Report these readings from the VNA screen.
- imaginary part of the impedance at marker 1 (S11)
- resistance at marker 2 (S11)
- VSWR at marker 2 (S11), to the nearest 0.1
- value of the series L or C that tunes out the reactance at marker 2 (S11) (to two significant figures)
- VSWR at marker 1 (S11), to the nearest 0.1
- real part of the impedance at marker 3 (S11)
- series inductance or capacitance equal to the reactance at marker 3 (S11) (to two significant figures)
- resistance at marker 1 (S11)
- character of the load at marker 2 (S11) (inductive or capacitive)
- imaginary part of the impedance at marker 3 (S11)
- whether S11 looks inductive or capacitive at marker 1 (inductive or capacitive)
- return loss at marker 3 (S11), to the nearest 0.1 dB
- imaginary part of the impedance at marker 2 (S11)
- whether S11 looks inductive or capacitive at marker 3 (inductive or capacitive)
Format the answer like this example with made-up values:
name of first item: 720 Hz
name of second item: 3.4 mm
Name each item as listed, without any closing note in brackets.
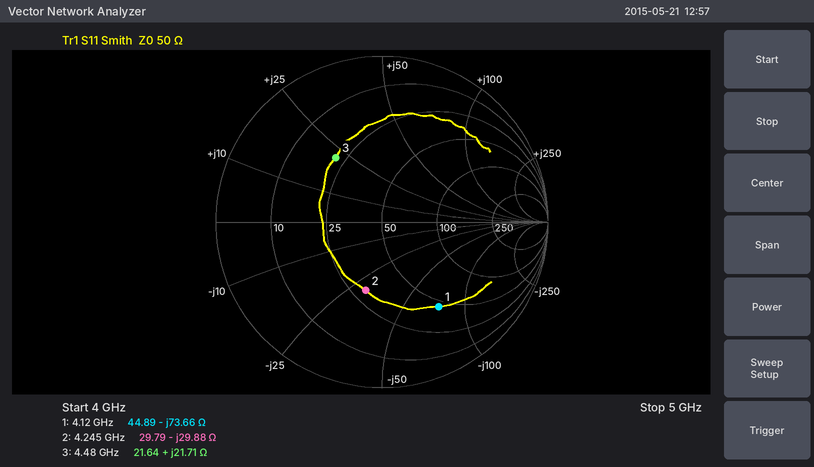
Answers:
imaginary part of the impedance at marker 1: -73.66 Ω
resistance at marker 2: 29.79 Ω
VSWR at marker 2 (S11), to the nearest 0.1: 2.5
value of the series L or C that tunes out the reactance at marker 2 (S11): 1.1 nH
VSWR at marker 1 (S11), to the nearest 0.1: 4.2
real part of the impedance at marker 3: 21.64 Ω
series inductance or capacitance equal to the reactance at marker 3 (S11): 770 pH
resistance at marker 1: 44.89 Ω
character of the load at marker 2 (S11): capacitive
imaginary part of the impedance at marker 3: +21.71 Ω
whether S11 looks inductive or capacitive at marker 1: capacitive
return loss at marker 3 (S11), to the nearest 0.1 dB: 6.4 dB
imaginary part of the impedance at marker 2: -29.88 Ω
whether S11 looks inductive or capacitive at marker 3: inductive
